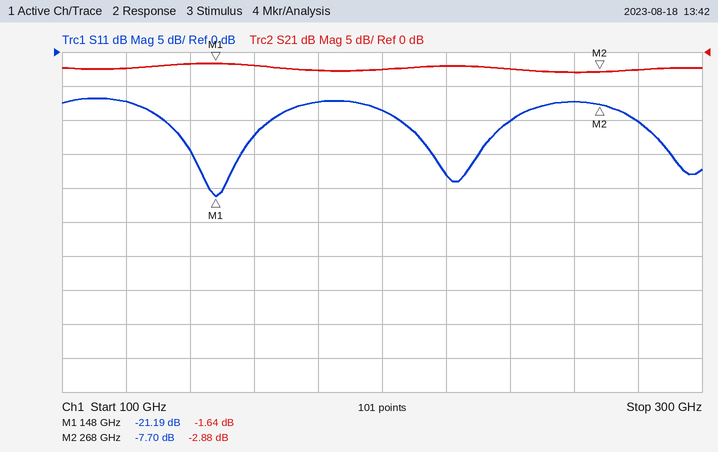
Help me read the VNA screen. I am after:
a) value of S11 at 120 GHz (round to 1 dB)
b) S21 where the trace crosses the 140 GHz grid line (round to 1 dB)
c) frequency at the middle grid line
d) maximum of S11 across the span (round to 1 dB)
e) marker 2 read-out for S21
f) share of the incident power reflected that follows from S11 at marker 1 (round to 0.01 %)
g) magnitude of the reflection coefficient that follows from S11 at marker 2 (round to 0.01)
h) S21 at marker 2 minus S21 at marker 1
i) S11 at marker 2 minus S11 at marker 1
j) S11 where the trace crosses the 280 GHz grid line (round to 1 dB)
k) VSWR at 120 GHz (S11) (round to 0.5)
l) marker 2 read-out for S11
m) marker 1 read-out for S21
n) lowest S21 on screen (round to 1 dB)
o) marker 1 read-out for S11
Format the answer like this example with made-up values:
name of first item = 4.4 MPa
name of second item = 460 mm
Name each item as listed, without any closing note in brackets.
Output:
value of S11 at 120 GHz = -7 dB
S21 where the trace crosses the 140 GHz grid line = -2 dB
frequency at the middle grid line = 200 GHz
maximum of S11 across the span = -7 dB
marker 2 read-out for S21 = -2.88 dB
share of the incident power reflected that follows from S11 at marker 1 = 0.76 %
magnitude of the reflection coefficient that follows from S11 at marker 2 = 0.41
S21 at marker 2 minus S21 at marker 1 = -1.24 dB
S11 at marker 2 minus S11 at marker 1 = 13.49 dB
S11 where the trace crosses the 280 GHz grid line = -10 dB
VSWR at 120 GHz (S11) = 2.5
marker 2 read-out for S11 = -7.70 dB
marker 1 read-out for S21 = -1.64 dB
lowest S21 on screen = -3 dB
marker 1 read-out for S11 = -21.19 dB
